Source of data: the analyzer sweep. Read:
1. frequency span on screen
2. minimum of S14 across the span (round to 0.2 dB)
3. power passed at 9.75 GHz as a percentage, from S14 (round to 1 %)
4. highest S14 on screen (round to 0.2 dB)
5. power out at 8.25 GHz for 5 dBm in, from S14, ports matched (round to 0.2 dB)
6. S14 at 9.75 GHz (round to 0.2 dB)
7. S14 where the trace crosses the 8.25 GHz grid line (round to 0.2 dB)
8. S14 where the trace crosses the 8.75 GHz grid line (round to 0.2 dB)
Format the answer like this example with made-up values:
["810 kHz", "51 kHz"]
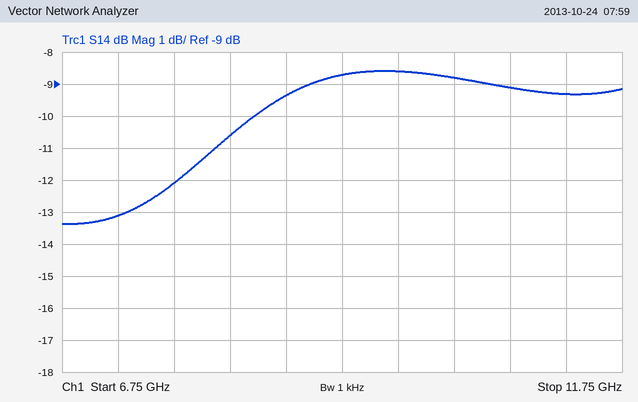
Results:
["5 GHz", "-13.4 dB", "14 %", "-8.6 dB", "-5.6 dBm", "-8.6 dB", "-10.6 dB", "-9.4 dB"]
